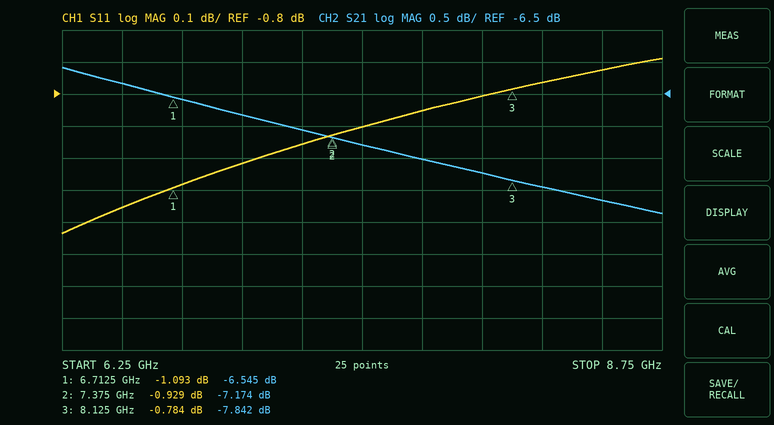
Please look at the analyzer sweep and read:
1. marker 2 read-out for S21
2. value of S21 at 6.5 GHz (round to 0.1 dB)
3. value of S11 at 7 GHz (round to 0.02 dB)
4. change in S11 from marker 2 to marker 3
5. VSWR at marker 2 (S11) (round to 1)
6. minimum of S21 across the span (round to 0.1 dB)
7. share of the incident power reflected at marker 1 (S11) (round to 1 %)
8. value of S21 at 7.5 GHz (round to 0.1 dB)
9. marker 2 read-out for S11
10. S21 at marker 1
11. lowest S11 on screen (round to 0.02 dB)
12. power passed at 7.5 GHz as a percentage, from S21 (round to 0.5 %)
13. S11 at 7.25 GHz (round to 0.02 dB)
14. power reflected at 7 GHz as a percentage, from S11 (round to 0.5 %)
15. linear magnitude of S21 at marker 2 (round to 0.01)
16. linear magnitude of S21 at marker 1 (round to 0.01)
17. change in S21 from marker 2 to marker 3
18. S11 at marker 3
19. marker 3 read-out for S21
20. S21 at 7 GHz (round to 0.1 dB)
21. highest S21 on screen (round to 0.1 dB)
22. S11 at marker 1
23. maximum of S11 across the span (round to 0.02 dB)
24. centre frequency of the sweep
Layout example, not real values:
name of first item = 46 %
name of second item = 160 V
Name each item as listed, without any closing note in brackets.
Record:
marker 2 read-out for S21 = -7.174 dB
value of S21 at 6.5 GHz = -6.3 dB
value of S11 at 7 GHz = -1.02 dB
change in S11 from marker 2 to marker 3 = 0.145 dB
VSWR at marker 2 (S11) = 19
minimum of S21 across the span = -8.4 dB
share of the incident power reflected at marker 1 (S11) = 78 %
value of S21 at 7.5 GHz = -7.3 dB
marker 2 read-out for S11 = -0.929 dB
S21 at marker 1 = -6.545 dB
lowest S11 on screen = -1.24 dB
power passed at 7.5 GHz as a percentage, from S21 = 18.5 %
S11 at 7.25 GHz = -0.96 dB
power reflected at 7 GHz as a percentage, from S11 = 79.0 %
linear magnitude of S21 at marker 2 = 0.44
linear magnitude of S21 at marker 1 = 0.47
change in S21 from marker 2 to marker 3 = -0.668 dB
S11 at marker 3 = -0.784 dB
marker 3 read-out for S21 = -7.842 dB
S21 at 7 GHz = -6.8 dB
highest S21 on screen = -6.1 dB
S11 at marker 1 = -1.093 dB
maximum of S11 across the span = -0.68 dB
centre frequency of the sweep = 7.5 GHz
